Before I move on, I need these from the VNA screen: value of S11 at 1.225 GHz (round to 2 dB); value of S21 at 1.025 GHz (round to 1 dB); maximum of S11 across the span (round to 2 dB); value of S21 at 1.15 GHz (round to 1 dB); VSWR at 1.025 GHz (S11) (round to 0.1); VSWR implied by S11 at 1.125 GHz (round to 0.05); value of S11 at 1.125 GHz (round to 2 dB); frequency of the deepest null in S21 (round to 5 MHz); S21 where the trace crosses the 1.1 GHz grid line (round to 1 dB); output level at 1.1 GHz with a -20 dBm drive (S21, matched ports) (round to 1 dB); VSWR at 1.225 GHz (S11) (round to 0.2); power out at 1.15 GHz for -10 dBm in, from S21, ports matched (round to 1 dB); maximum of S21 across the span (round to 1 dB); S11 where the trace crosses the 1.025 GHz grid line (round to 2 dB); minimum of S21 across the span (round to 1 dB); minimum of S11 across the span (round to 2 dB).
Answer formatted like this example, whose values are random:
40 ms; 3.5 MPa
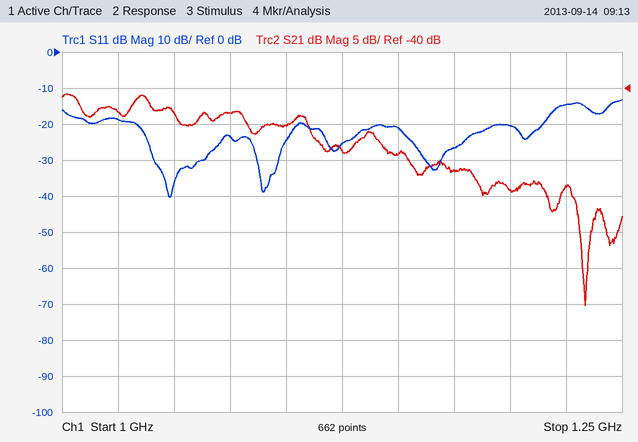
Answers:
-14 dB; -43 dB; -14 dB; -49 dB; 1.3; 1.10; -26 dB; 1.235 GHz; -45 dB; -65 dBm; 1.4; -59 dBm; -41 dB; -18 dB; -70 dB; -40 dB
